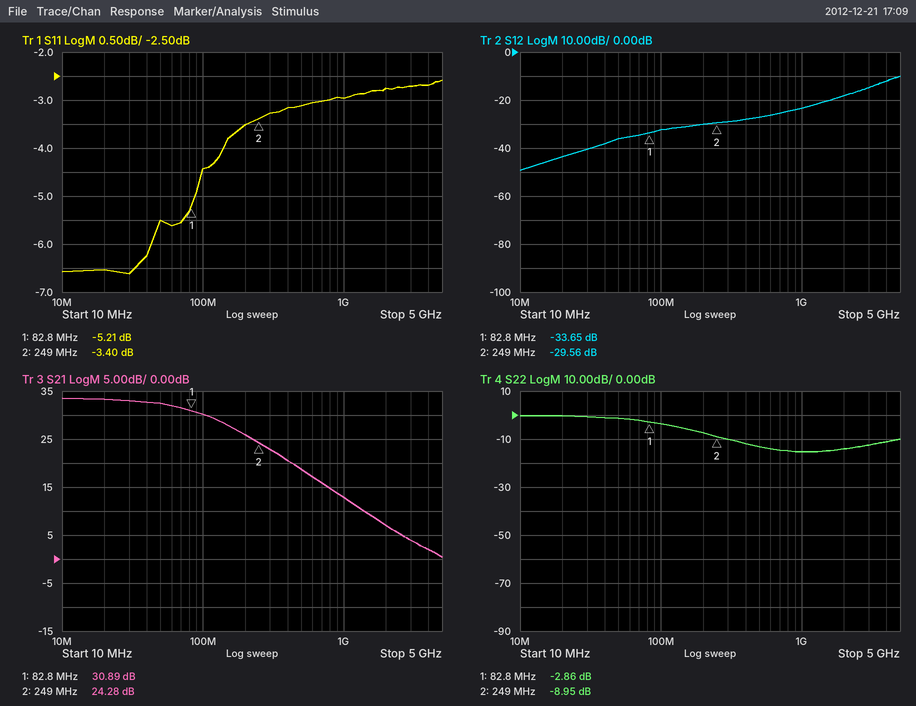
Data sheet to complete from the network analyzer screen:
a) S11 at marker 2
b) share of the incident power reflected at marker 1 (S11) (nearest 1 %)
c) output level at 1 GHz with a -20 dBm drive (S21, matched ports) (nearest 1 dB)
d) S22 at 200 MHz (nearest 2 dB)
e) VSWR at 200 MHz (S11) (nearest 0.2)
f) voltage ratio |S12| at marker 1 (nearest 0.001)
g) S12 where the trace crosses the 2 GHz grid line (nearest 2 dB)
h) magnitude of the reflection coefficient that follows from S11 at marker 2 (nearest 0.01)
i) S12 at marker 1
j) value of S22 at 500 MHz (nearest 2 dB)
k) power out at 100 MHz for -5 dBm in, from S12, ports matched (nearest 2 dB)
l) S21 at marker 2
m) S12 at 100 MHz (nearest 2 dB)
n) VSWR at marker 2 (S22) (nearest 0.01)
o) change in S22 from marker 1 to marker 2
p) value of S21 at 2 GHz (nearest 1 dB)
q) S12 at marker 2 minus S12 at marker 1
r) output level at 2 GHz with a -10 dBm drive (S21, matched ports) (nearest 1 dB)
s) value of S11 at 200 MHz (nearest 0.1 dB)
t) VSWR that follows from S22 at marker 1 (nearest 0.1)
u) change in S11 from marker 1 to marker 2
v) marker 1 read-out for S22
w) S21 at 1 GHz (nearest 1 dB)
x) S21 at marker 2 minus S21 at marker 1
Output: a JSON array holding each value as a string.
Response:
["-3.40 dB", "30 %", "-7 dBm", "-8 dB", "5.0", "0.021", "-18 dB", "0.68", "-33.65 dB", "-14 dB", "-38 dBm", "24.28 dB", "-32 dB", "2.11", "-6.09 dB", "7 dB", "4.09 dB", "-3 dBm", "-3.5 dB", "6.1", "1.81 dB", "-2.86 dB", "13 dB", "-6.61 dB"]
